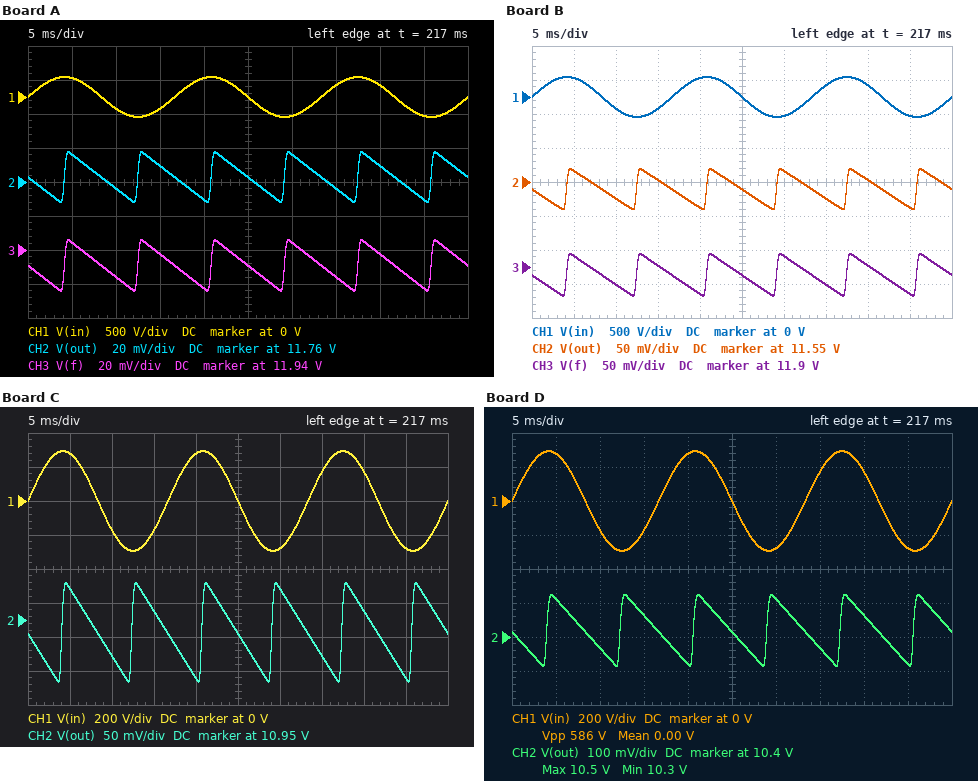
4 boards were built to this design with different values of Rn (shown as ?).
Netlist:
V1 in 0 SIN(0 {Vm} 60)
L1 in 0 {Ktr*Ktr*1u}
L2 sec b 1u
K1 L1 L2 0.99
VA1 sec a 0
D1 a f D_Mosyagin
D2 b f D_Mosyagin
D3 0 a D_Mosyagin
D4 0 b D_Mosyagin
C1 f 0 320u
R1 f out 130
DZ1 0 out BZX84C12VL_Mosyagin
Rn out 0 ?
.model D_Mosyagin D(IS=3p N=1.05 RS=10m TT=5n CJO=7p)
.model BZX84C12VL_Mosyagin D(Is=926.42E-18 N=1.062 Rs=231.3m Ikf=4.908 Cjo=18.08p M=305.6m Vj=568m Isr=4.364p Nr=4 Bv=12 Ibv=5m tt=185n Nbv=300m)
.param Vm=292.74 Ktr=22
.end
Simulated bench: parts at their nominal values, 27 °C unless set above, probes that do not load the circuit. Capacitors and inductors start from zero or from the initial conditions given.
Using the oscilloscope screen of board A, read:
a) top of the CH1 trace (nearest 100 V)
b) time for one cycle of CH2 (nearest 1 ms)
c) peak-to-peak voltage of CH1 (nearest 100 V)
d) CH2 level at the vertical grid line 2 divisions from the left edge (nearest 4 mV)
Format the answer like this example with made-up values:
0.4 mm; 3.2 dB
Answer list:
300 V; 8 ms; 600 V; 11.756 V
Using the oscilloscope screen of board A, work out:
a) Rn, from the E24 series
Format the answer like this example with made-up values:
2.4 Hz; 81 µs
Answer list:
9.1 kΩ
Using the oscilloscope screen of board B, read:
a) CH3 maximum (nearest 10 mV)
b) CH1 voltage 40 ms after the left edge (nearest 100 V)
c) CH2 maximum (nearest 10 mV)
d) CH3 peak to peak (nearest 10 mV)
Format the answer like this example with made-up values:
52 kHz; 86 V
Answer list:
11.92 V; 200 V; 11.57 V; 60 mV
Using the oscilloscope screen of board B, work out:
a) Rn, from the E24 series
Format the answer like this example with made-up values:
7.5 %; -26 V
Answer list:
4.3 kΩ
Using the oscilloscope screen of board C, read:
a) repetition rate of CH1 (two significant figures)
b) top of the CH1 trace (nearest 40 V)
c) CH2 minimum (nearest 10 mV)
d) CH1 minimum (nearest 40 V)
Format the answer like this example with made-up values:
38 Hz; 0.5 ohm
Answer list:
60 Hz; 280 V; 10.86 V; -280 V
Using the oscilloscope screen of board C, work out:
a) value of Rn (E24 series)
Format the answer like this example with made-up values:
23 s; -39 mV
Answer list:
1.6 kΩ
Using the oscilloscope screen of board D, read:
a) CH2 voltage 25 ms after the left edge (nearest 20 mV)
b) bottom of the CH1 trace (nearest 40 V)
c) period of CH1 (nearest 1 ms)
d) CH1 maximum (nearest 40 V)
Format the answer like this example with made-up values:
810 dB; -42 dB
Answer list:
10.42 V; -280 V; 17 ms; 280 V
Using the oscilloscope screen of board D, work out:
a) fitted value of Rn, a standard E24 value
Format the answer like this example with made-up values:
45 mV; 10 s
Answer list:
1 kΩ
